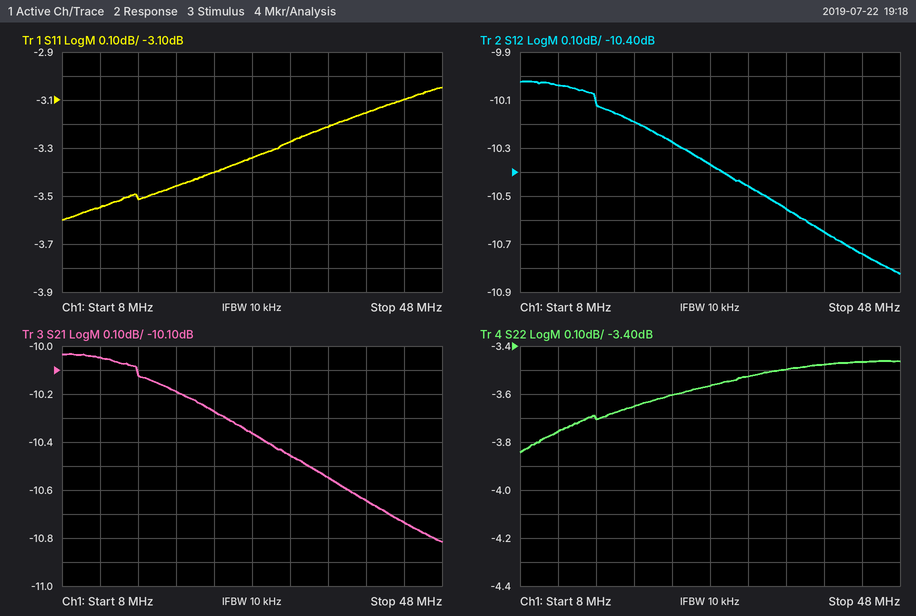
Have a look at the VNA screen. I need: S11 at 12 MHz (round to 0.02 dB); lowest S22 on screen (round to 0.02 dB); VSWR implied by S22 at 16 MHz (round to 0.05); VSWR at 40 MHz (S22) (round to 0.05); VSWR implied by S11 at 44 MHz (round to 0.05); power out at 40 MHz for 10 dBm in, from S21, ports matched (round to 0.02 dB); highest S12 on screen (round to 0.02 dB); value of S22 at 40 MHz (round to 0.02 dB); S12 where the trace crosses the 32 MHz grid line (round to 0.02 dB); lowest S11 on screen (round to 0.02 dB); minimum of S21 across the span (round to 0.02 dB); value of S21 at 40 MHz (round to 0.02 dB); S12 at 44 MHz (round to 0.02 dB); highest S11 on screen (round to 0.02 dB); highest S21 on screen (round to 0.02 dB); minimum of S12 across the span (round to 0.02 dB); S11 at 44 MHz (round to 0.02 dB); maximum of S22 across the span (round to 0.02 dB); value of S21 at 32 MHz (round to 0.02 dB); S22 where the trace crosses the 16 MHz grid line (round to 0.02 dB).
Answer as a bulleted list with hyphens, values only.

- -3.54 dB
- -3.84 dB
- 4.75
- 5.05
- 5.65
- -0.64 dBm
- -10.02 dB
- -3.48 dB
- -10.46 dB
- -3.60 dB
- -10.82 dB
- -10.64 dB
- -10.74 dB
- -3.04 dB
- -10.04 dB
- -10.82 dB
- -3.10 dB
- -3.46 dB
- -10.46 dB
- -3.70 dB
